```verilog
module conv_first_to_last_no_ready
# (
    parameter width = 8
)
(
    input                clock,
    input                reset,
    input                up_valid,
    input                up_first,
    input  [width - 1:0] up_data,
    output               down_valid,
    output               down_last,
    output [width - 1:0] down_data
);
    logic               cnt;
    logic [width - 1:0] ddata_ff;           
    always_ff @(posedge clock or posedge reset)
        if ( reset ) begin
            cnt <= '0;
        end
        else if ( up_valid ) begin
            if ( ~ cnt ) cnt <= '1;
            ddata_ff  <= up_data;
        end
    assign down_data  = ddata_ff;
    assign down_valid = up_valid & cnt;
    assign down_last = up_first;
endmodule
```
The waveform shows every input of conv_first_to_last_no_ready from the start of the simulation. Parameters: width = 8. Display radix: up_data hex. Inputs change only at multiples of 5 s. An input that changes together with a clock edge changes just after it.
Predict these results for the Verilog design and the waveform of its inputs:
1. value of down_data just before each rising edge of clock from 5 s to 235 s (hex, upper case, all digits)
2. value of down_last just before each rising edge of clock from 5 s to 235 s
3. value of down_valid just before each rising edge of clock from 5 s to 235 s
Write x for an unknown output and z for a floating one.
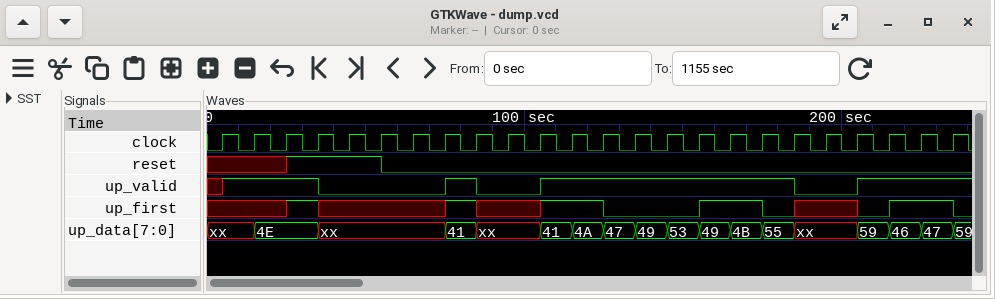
x, x, x, 4E, 4E, 4E, 4E, 4E, 4E, 41, 41, 41, 41, 4A, 47, 49, 53, 49, 4B, 55, 55, 55, 59, 46
x x x 1 x x x x 1 x x 1 1 0 0 0 1 1 0 x x 0 1 1
x x x 0 0 0 0 0 0 0 0 1 1 1 1 1 1 1 1 0 0 1 1 1
